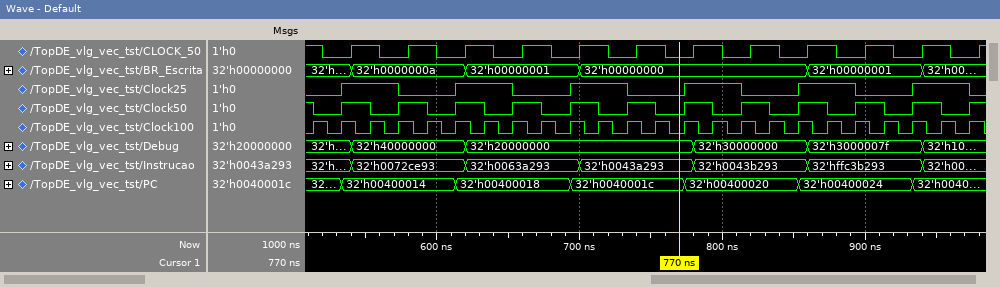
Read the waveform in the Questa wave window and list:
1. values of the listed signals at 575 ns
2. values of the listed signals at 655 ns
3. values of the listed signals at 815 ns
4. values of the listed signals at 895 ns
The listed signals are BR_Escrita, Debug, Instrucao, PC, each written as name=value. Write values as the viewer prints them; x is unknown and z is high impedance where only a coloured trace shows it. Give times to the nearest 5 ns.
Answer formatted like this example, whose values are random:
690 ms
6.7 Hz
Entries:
BR_Escrita=32'h0000000a, Debug=32'h40000000, Instrucao=32'h0072ce93, PC=32'h00400014
BR_Escrita=32'h00000001, Debug=32'h20000000, Instrucao=32'h0063a293, PC=32'h00400018
BR_Escrita=32'h00000000, Debug=32'h30000000, Instrucao=32'h0043b293, PC=32'h00400020
BR_Escrita=32'h00000001, Debug=32'h3000007f, Instrucao=32'hffc3b293, PC=32'h00400024
